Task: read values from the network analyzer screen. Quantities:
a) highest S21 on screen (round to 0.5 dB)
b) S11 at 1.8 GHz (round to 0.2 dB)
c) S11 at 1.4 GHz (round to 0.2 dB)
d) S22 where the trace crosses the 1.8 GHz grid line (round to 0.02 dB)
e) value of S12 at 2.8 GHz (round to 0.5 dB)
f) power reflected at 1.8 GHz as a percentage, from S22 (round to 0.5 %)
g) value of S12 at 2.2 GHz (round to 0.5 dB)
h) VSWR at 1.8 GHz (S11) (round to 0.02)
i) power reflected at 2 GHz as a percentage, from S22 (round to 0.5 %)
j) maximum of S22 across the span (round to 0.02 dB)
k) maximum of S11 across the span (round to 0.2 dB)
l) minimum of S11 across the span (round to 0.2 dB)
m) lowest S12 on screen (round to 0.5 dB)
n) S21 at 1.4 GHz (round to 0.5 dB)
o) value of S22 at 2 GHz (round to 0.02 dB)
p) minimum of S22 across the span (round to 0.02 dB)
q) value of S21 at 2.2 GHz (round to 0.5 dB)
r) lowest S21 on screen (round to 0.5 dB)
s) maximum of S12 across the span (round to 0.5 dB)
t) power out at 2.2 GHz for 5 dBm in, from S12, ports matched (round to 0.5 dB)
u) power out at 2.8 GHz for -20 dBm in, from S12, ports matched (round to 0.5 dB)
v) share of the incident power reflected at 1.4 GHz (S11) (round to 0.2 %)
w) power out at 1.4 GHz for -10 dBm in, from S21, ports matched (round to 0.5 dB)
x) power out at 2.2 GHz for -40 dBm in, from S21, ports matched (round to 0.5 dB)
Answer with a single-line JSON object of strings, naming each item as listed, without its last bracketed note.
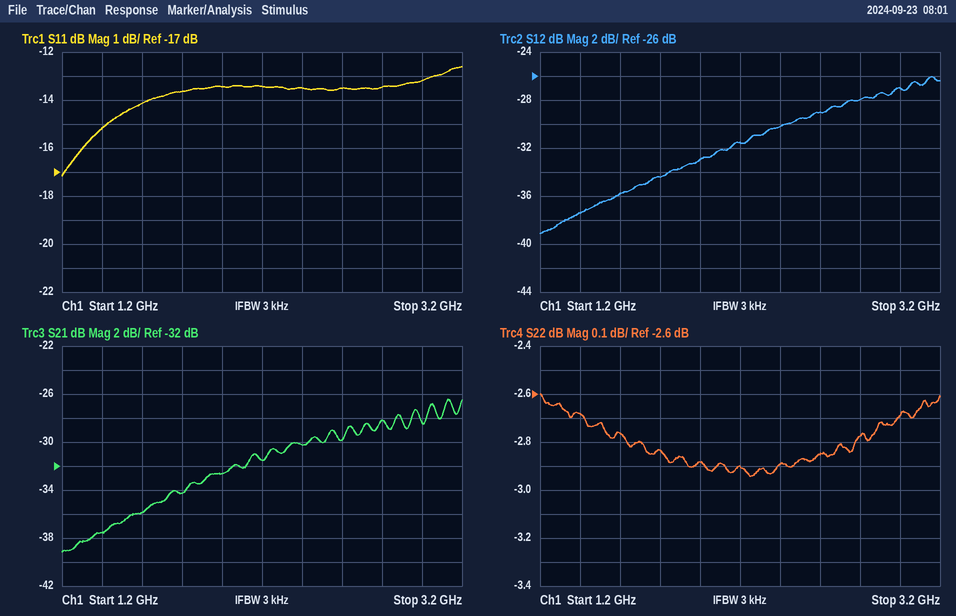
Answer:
{"highest S21 on screen": "-26.5 dB", "S11 at 1.8 GHz": "-13.6 dB", "S11 at 1.4 GHz": "-15.2 dB", "S22 where the trace crosses the 1.8 GHz grid line": "-2.84 dB", "value of S12 at 2.8 GHz": "-28.0 dB", "power reflected at 1.8 GHz as a percentage, from S22": "52.0 %", "value of S12 at 2.2 GHz": "-31.5 dB", "VSWR at 1.8 GHz (S11)": "1.52", "power reflected at 2 GHz as a percentage, from S22": "51.5 %", "maximum of S22 across the span": "-2.60 dB", "maximum of S11 across the span": "-12.6 dB", "minimum of S11 across the span": "-17.2 dB", "lowest S12 on screen": "-39.0 dB", "S21 at 1.4 GHz": "-37.5 dB", "value of S22 at 2 GHz": "-2.88 dB", "minimum of S22 across the span": "-2.94 dB", "value of S21 at 2.2 GHz": "-31.5 dB", "lowest S21 on screen": "-39.0 dB", "maximum of S12 across the span": "-26.0 dB", "power out at 2.2 GHz for 5 dBm in, from S12, ports matched": "-26.5 dBm", "power out at 2.8 GHz for -20 dBm in, from S12, ports matched": "-48.0 dBm", "share of the incident power reflected at 1.4 GHz (S11)": "3.0 %", "power out at 1.4 GHz for -10 dBm in, from S21, ports matched": "-47.5 dBm", "power out at 2.2 GHz for -40 dBm in, from S21, ports matched": "-71.5 dBm"}
